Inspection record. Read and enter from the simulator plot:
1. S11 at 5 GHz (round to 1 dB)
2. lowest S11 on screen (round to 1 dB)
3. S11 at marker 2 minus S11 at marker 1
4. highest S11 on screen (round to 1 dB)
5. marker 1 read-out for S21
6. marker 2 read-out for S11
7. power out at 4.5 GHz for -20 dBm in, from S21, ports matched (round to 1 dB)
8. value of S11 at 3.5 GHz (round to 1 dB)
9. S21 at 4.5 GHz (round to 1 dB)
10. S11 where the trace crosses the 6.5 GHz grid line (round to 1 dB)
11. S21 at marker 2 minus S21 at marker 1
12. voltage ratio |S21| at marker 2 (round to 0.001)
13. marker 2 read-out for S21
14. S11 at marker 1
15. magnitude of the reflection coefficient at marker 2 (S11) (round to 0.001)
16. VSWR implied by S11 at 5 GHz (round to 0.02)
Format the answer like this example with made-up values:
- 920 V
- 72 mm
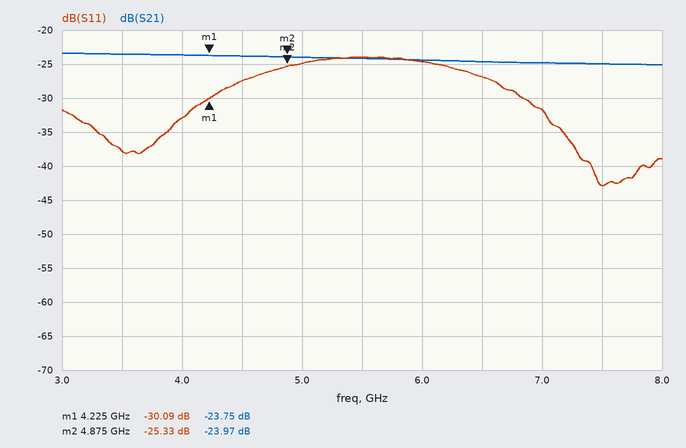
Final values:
- -25 dB
- -43 dB
- 4.76 dB
- -24 dB
- -23.75 dB
- -25.33 dB
- -44 dBm
- -38 dB
- -24 dB
- -27 dB
- -0.22 dB
- 0.063
- -23.97 dB
- -30.09 dB
- 0.054
- 1.12
